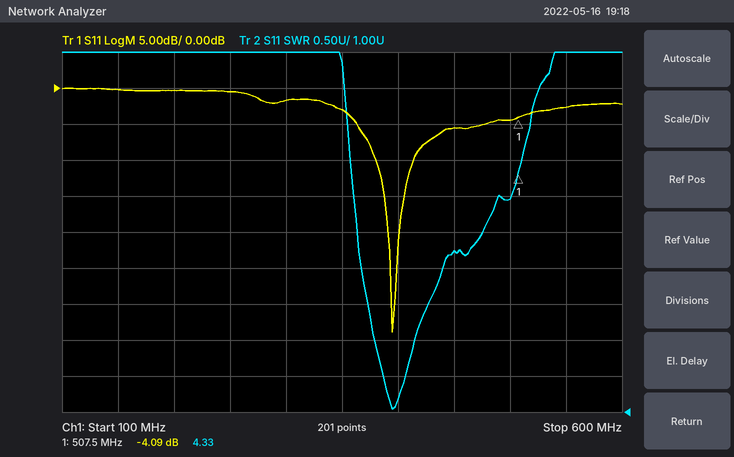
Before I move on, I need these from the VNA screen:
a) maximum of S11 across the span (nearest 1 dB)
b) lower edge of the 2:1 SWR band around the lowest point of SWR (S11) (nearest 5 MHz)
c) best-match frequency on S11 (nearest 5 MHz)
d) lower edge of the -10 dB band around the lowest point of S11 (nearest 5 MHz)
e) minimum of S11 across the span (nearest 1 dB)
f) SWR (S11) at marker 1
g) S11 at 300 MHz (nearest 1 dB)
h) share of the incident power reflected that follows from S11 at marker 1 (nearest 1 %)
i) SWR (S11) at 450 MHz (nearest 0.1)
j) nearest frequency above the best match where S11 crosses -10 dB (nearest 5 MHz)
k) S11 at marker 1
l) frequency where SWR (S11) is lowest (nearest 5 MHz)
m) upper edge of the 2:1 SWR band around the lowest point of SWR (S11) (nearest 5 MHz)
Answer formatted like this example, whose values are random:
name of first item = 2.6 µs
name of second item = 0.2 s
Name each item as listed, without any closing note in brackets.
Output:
maximum of S11 across the span = 0 dB
lower edge of the 2:1 SWR band around the lowest point of SWR (S11) = 380 MHz
best-match frequency on S11 = 395 MHz
lower edge of the -10 dB band around the lowest point of S11 = 380 MHz
minimum of S11 across the span = -34 dB
SWR (S11) at marker 1 = 4.33
S11 at 300 MHz = -2 dB
share of the incident power reflected that follows from S11 at marker 1 = 39 %
SWR (S11) at 450 MHz = 3.2
nearest frequency above the best match where S11 crosses -10 dB = 415 MHz
S11 at marker 1 = -4.09 dB
frequency where SWR (S11) is lowest = 395 MHz
upper edge of the 2:1 SWR band around the lowest point of SWR (S11) = 415 MHz
